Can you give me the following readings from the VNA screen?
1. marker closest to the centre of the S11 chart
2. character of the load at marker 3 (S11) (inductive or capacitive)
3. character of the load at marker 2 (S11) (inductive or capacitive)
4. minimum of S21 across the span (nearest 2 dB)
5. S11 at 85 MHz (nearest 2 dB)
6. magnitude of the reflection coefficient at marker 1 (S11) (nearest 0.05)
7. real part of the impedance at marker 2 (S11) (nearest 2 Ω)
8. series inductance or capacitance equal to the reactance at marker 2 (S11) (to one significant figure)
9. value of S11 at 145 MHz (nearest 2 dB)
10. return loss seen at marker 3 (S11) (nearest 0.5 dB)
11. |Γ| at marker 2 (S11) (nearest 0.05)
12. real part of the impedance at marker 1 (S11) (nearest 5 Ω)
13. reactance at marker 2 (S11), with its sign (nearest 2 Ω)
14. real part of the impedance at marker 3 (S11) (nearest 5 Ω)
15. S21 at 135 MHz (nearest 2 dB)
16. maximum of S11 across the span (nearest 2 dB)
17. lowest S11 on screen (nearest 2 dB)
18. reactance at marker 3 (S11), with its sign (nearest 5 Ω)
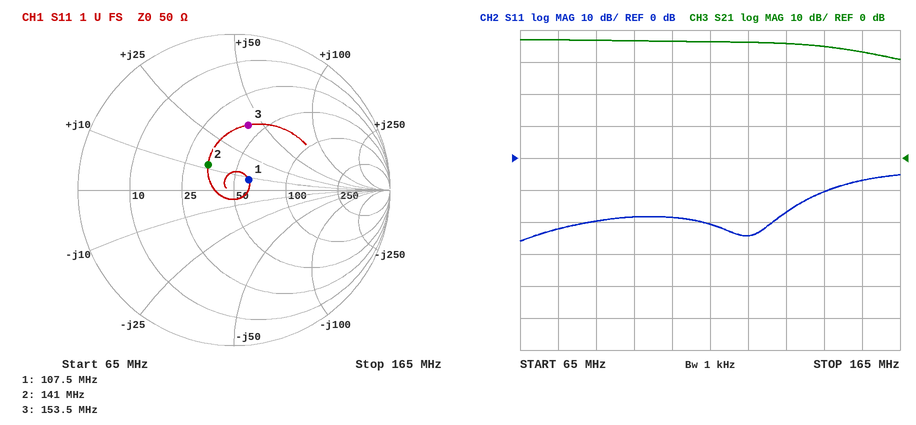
marker 1
inductive
inductive
30 dB
-20 dB
0.10
34 Ω
10 nH
-10 dB
7.5 dB
0.25
60 Ω
+12 Ω
40 Ω
36 dB
-6 dB
-26 dB
+40 Ω
